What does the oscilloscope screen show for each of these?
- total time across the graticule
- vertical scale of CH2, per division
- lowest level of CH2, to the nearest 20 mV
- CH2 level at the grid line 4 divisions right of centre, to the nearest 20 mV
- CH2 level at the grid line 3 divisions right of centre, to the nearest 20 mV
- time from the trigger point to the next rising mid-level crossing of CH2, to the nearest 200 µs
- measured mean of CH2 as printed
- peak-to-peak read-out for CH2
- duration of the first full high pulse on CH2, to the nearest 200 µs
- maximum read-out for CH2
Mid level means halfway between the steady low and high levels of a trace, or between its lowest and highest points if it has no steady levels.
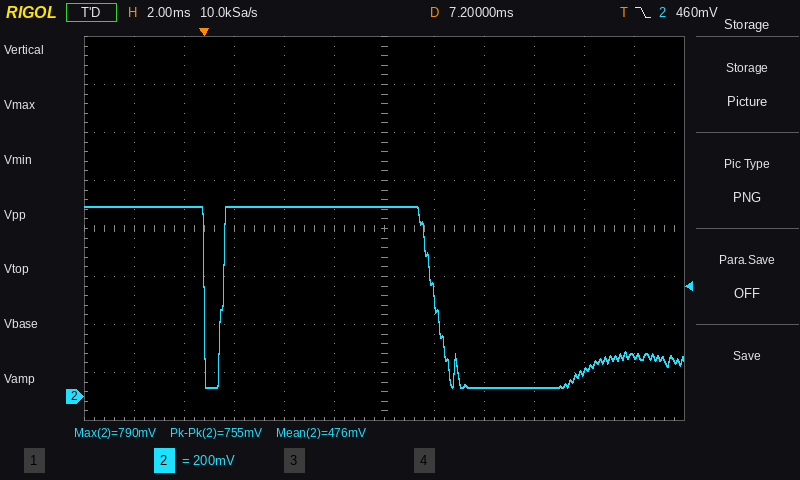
24 ms
200 mV
40 mV
100 mV
40 mV
800 µs
476 mV
755 mV
8.4 ms
790 mV
